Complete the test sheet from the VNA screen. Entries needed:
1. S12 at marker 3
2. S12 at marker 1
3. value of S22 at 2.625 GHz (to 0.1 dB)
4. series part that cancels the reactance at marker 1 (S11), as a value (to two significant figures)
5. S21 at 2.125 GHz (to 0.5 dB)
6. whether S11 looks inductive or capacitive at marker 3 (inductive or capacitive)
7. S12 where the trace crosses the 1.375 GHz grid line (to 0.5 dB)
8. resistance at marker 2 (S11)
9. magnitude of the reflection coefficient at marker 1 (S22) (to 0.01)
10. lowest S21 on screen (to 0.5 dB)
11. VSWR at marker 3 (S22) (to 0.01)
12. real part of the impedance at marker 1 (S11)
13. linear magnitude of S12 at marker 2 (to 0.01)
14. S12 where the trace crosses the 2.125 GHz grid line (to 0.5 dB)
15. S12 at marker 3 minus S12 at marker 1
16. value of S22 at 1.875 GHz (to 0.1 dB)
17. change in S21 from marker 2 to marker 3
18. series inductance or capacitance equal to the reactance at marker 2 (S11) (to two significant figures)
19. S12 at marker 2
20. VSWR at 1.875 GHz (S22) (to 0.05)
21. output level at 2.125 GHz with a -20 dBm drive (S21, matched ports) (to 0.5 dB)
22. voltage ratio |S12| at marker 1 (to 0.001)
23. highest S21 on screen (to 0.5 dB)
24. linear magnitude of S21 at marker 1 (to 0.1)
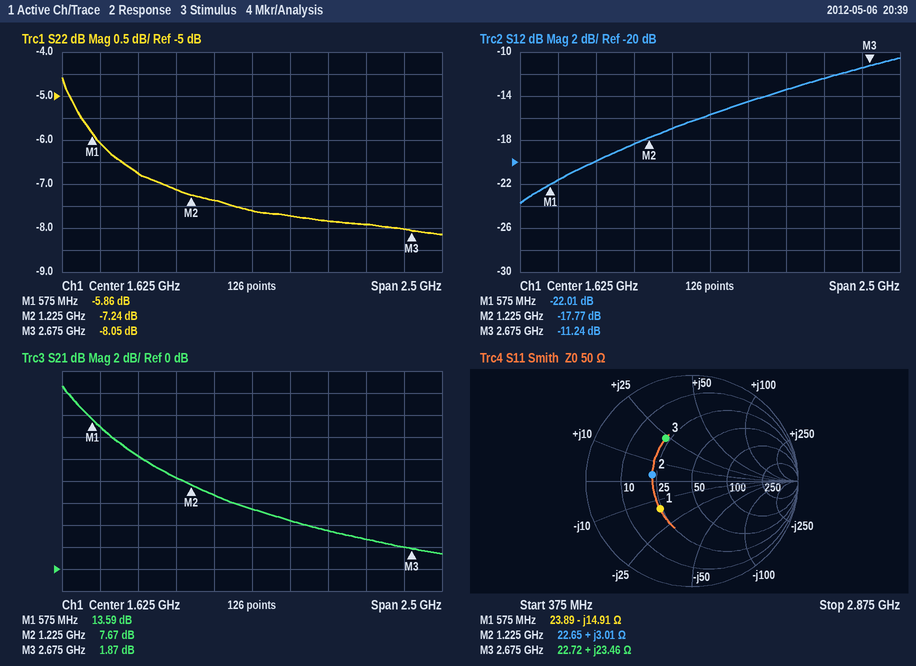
-11.24 dB
-22.01 dB
-8.0 dB
4.1 nH
3.5 dB
inductive
-17.0 dB
22.65 Ω
0.51
1.5 dB
2.31
23.89 Ω
0.13
-13.5 dB
10.77 dB
-7.7 dB
-5.80 dB
390 pH
-17.77 dB
2.40
-16.5 dBm
0.079
16.5 dB
4.8
